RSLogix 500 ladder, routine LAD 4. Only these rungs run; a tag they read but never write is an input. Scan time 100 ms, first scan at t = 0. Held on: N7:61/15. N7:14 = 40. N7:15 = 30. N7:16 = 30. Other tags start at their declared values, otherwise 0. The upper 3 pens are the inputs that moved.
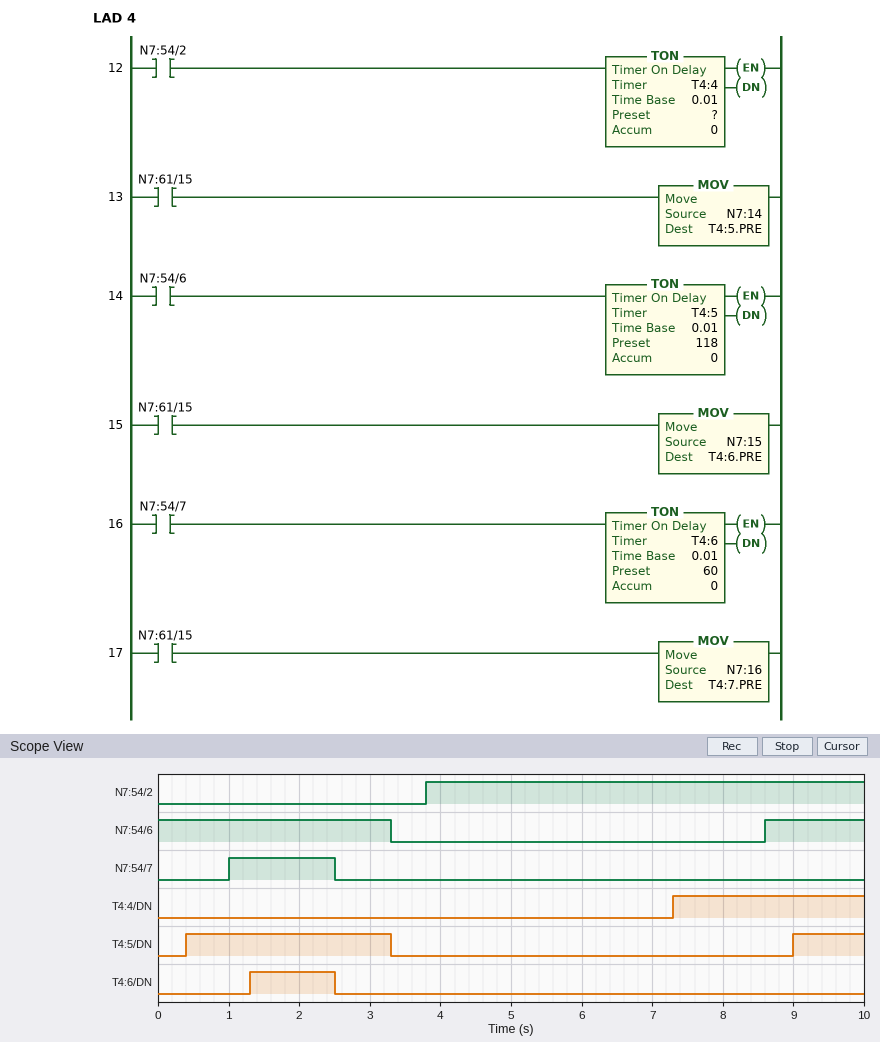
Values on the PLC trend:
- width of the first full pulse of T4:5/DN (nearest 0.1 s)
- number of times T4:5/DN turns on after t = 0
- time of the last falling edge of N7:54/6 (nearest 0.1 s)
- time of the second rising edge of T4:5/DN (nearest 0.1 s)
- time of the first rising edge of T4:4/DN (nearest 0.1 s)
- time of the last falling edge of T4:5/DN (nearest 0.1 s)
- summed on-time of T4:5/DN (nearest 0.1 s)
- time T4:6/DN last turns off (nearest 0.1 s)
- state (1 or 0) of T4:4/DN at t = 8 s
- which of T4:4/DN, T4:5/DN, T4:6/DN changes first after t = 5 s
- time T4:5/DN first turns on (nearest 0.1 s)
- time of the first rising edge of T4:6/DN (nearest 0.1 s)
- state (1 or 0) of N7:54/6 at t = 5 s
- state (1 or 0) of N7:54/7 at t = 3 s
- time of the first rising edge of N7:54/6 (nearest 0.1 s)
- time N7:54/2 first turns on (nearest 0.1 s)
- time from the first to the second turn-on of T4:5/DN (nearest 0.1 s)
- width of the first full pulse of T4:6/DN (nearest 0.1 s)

2.9 s
2
3.3 s
9.0 s
7.3 s
3.3 s
3.9 s
2.5 s
1
T4:4/DN
0.4 s
1.3 s
0
0
8.6 s
3.8 s
8.6 s
1.2 s
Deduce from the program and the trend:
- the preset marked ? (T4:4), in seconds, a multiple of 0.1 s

3.5 s
